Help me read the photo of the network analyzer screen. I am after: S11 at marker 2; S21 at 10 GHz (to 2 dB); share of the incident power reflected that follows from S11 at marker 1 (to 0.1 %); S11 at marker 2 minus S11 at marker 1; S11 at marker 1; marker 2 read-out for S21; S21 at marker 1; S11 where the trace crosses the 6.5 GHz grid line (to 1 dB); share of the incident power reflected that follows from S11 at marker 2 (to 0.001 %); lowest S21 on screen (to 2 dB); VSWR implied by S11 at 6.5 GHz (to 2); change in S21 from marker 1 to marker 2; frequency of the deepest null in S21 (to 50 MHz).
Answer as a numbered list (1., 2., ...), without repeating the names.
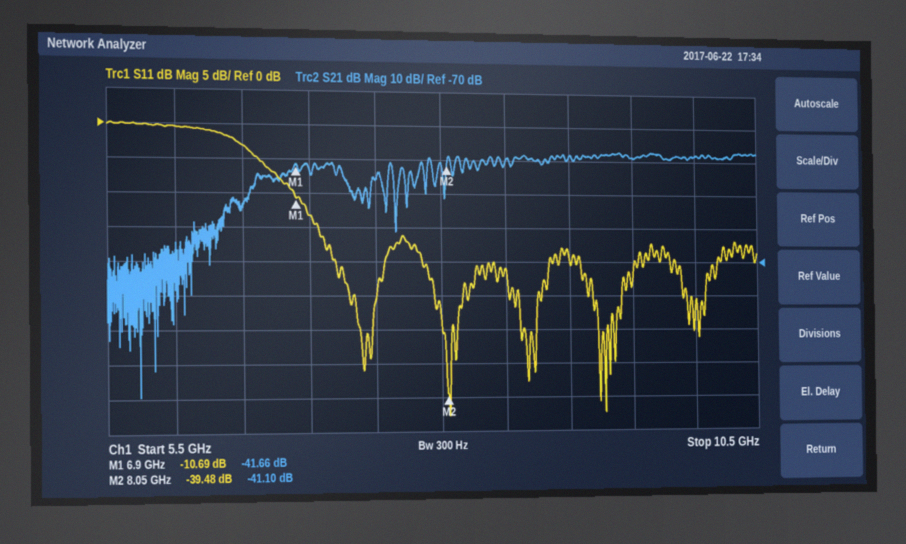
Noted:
1. -39.48 dB
2. -38 dB
3. 8.5 %
4. -28.79 dB
5. -10.69 dB
6. -41.10 dB
7. -41.66 dB
8. -3 dB
9. 0.011 %
10. -110 dB
11. 6
12. 0.56 dB
13. 5.75 GHz
